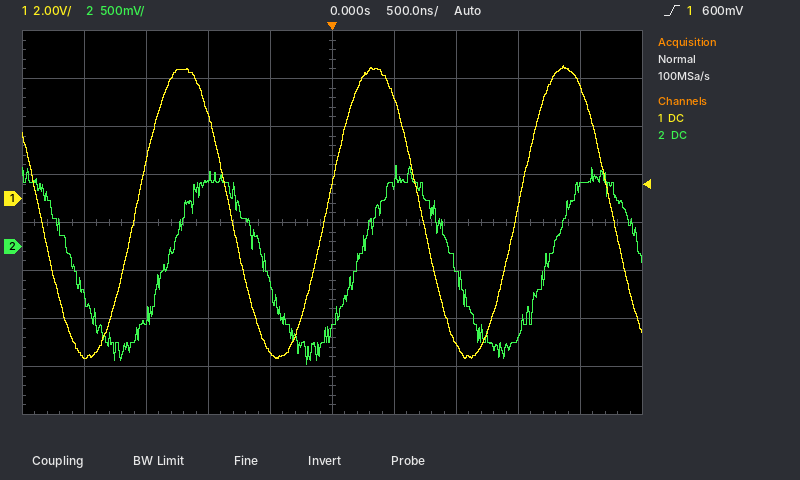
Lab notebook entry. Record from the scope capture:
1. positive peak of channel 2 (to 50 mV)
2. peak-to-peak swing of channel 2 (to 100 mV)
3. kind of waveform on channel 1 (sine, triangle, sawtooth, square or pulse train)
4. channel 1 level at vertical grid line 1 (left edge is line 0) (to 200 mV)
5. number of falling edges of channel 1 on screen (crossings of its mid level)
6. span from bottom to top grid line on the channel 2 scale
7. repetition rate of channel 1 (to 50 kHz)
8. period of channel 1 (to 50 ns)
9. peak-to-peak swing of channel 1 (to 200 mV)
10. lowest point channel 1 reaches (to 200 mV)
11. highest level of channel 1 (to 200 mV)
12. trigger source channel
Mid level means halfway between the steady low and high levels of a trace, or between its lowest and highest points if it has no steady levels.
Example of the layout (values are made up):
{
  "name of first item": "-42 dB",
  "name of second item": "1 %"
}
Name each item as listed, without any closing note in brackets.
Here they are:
{
  "positive peak of channel 2": "850 mV",
  "peak-to-peak swing of channel 2": "2.10 V",
  "kind of waveform on channel 1": "sine",
  "channel 1 level at vertical grid line 1 (left edge is line 0)": "-6.6 V",
  "number of falling edges of channel 1 on screen": "4",
  "span from bottom to top grid line on the channel 2 scale": "4 V",
  "repetition rate of channel 1": "650 kHz",
  "period of channel 1": "1.55 µs",
  "peak-to-peak swing of channel 1": "12.2 V",
  "lowest point channel 1 reaches": "-6.6 V",
  "highest level of channel 1": "5.6 V",
  "trigger source channel": "channel 1"
}
